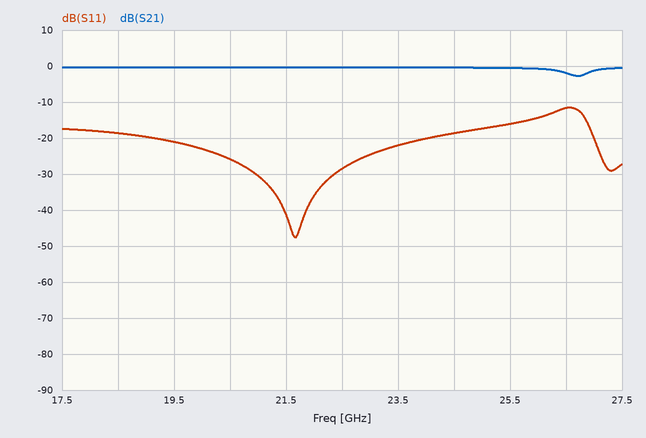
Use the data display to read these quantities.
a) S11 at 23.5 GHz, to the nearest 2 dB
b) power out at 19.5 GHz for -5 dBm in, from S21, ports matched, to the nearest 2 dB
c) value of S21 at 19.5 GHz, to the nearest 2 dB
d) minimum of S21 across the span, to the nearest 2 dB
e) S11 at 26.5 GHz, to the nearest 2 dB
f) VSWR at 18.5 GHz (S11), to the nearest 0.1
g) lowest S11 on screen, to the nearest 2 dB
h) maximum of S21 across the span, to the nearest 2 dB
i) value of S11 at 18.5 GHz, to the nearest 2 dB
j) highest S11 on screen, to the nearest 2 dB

-22 dB
-6 dBm
0 dB
-2 dB
-12 dB
1.3
-48 dB
0 dB
-18 dB
-12 dB
